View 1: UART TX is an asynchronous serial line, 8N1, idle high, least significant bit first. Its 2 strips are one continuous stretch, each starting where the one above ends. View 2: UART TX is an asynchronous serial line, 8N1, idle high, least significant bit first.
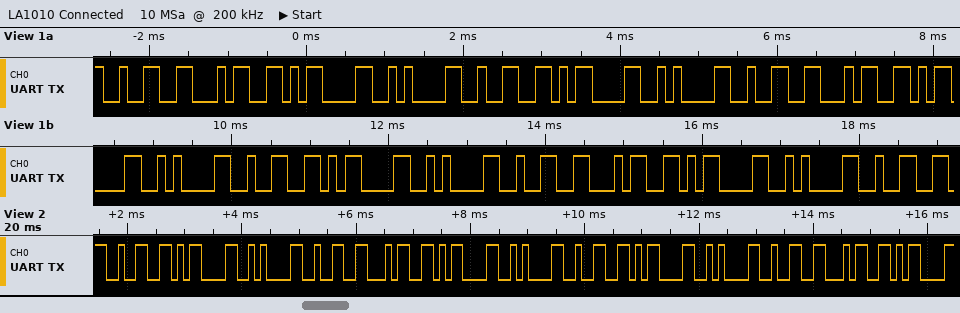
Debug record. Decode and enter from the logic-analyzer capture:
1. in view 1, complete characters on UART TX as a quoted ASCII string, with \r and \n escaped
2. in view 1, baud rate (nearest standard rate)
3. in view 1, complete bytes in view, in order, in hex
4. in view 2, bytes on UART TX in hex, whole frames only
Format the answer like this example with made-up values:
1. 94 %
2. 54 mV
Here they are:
1. "24\r\n2\r\n24\r\n2\r\n24\r\n2"
2. 9600 baud
3. 32 34 0D 0A 32 0D 0A 32 34 0D 0A 32 0D 0A 32 34 0D 0A 32
4. 32 0D 0A 32 34 0D 0A 32 0D 0A 32 34 0D
